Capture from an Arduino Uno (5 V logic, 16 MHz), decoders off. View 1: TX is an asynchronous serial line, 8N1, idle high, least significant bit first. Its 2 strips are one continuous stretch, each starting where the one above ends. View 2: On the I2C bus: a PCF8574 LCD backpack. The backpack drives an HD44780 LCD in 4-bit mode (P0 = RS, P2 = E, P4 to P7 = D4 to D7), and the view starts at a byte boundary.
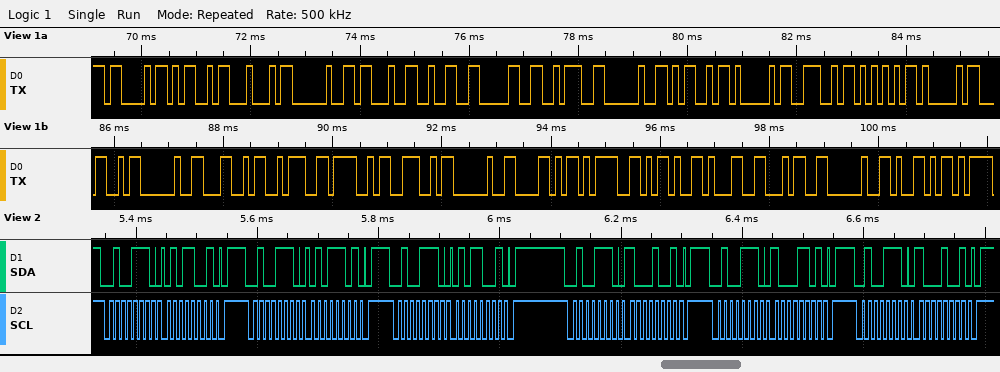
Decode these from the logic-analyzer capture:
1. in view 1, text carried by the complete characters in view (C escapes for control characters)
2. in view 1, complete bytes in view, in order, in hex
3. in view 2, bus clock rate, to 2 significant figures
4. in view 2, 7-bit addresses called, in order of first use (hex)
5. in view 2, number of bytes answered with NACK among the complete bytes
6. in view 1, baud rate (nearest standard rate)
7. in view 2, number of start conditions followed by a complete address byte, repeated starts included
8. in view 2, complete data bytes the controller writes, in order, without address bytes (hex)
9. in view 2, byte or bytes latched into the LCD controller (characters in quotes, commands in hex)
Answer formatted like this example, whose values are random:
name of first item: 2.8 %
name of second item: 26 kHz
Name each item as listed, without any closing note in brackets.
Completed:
in view 1, text carried by the complete characters in view: "CMD #20: MANUAL L:ON X=-14 Y"
in view 1, complete bytes in view, in order, in hex: 0x43 0x4D 0x44 0x20 0x23 0x32 0x30 0x3A 0x20 0x4D 0x41 0x4E 0x55 0x41 0x4C 0x20 0x4C 0x3A 0x4F 0x4E 0x20 0x58 0x3D 0x2D 0x31 0x34 0x20 0x59
in view 2, bus clock rate, to 2 significant figures: 100 kHz
in view 2, 7-bit addresses called, in order of first use: 0x27
in view 2, number of bytes answered with NACK among the complete bytes: 0
in view 1, baud rate: 9600 baud
in view 2, number of start conditions followed by a complete address byte, repeated starts included: 6
in view 2, complete data bytes the controller writes, in order, without address bytes: 59 5D 59 89 8D 89
in view 2, byte or bytes latched into the LCD controller: 'X'
